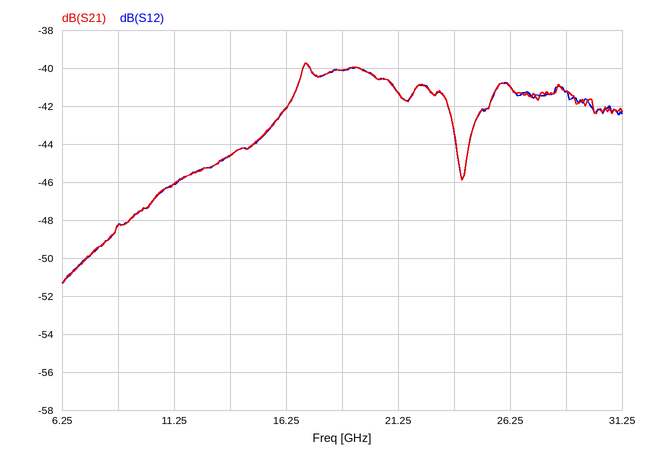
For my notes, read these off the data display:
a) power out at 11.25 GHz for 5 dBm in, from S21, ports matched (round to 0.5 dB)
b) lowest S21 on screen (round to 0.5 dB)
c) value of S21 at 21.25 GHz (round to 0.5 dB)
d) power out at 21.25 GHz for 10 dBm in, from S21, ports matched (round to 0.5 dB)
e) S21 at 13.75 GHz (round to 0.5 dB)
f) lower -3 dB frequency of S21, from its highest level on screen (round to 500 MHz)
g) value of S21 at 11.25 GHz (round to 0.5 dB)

-41.0 dBm
-51.5 dB
-41.5 dB
-31.5 dBm
-44.5 dB
16.0 GHz
-46.0 dB
